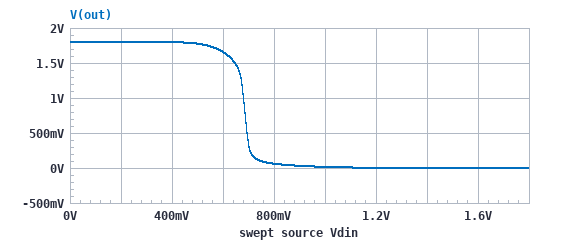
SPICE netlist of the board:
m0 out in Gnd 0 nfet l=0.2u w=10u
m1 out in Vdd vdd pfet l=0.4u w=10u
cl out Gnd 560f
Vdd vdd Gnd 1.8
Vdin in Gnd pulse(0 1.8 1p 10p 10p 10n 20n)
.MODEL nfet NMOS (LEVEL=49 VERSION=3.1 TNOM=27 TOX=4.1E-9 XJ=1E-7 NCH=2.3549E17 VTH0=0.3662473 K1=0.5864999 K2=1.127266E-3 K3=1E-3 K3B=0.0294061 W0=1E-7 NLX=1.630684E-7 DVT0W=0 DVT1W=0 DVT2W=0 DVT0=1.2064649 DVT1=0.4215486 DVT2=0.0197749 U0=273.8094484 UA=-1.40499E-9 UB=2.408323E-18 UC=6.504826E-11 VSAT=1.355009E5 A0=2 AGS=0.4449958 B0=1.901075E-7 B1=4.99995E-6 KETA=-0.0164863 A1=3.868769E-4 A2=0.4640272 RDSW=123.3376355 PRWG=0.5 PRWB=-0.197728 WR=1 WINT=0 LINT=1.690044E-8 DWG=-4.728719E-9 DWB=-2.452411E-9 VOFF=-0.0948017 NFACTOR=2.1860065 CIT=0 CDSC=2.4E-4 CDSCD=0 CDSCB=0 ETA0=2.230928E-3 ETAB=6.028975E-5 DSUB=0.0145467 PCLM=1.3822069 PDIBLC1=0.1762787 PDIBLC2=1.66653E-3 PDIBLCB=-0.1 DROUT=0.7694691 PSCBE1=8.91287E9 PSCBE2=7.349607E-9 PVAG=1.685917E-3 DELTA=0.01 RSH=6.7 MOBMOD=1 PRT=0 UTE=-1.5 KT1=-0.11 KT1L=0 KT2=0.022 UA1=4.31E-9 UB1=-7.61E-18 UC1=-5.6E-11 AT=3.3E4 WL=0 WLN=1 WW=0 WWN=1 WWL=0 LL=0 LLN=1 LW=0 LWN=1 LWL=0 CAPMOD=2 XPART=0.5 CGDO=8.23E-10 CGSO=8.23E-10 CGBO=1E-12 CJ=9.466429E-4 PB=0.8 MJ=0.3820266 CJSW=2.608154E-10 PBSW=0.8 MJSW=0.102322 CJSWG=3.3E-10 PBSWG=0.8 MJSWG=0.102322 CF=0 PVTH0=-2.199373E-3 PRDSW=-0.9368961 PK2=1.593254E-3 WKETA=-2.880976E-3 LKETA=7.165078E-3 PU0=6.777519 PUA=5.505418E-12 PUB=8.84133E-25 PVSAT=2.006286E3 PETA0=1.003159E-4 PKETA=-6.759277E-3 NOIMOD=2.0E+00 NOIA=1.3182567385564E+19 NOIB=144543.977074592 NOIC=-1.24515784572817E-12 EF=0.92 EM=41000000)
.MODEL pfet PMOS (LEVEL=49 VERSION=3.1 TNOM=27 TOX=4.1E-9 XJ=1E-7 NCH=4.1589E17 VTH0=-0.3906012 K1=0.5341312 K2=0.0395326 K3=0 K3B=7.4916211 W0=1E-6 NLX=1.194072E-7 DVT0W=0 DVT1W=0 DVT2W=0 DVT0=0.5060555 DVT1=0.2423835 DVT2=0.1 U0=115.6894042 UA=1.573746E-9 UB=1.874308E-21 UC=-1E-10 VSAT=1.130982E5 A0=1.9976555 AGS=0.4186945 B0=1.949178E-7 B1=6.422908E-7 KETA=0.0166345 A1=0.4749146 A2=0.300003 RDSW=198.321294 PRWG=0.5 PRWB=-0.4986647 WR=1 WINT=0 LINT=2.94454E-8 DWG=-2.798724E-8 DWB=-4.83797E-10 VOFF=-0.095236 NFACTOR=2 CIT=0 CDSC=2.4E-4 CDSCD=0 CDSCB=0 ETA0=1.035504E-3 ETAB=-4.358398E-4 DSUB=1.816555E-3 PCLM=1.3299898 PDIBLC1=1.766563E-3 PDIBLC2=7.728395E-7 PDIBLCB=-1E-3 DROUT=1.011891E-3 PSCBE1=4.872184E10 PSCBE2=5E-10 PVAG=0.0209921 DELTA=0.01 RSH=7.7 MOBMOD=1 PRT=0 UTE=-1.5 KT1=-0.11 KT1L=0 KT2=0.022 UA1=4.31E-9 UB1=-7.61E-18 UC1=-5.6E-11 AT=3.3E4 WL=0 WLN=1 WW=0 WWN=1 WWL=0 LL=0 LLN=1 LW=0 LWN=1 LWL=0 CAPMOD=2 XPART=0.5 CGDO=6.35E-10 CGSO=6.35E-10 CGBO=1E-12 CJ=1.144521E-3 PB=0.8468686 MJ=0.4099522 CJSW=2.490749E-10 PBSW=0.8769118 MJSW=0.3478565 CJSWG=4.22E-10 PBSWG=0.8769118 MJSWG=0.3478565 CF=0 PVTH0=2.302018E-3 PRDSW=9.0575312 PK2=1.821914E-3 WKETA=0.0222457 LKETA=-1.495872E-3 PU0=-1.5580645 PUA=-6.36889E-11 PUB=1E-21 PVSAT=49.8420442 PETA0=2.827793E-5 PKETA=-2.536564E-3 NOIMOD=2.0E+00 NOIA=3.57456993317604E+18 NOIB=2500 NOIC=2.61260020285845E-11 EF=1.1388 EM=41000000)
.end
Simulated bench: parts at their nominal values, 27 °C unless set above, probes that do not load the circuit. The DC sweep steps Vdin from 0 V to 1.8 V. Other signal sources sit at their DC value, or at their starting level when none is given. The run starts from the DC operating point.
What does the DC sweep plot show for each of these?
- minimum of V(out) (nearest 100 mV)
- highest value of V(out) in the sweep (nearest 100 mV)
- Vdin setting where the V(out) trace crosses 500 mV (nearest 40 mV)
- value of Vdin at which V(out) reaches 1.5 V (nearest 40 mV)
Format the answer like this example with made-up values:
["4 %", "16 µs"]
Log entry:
["0 V", "1.8 V", "680 mV", "640 mV"]
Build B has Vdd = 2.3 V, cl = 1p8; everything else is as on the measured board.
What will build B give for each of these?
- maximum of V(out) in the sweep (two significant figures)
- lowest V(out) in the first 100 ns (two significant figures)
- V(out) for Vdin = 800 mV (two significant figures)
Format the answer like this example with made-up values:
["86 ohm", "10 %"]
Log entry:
["2.3 V", "-24 mV", "960 mV"]
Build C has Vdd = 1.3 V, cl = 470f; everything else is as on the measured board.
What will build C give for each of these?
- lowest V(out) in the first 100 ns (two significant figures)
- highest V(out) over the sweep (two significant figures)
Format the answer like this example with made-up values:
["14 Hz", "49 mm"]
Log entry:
["-84 mV", "1.3 V"]
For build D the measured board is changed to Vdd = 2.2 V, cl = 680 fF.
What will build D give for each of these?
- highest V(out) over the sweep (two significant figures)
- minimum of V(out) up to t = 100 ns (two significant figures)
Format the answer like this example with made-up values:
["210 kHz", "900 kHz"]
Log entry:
["2.2 V", "-64 mV"]
